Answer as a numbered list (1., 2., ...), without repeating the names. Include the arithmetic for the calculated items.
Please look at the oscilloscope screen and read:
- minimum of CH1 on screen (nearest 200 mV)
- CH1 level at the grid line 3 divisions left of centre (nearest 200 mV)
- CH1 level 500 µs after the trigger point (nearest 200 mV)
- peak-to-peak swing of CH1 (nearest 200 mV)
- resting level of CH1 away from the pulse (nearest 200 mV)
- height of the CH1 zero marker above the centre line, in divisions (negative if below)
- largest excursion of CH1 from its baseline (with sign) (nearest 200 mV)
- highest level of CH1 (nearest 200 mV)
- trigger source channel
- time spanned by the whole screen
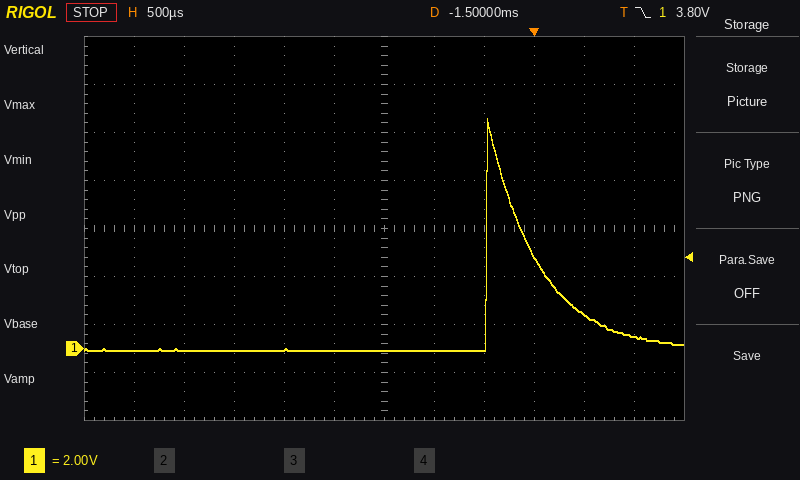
1. 0.0 V
2. 0.0 V
3. 1.4 V
4. 9.6 V − (0.0 V) = 9.6 V
5. 0.0 V
6. -2.5 div
7. 9.6 V − (0.0 V) = +9.6 V
8. 9.6 V
9. CH1
10. 6 ms
